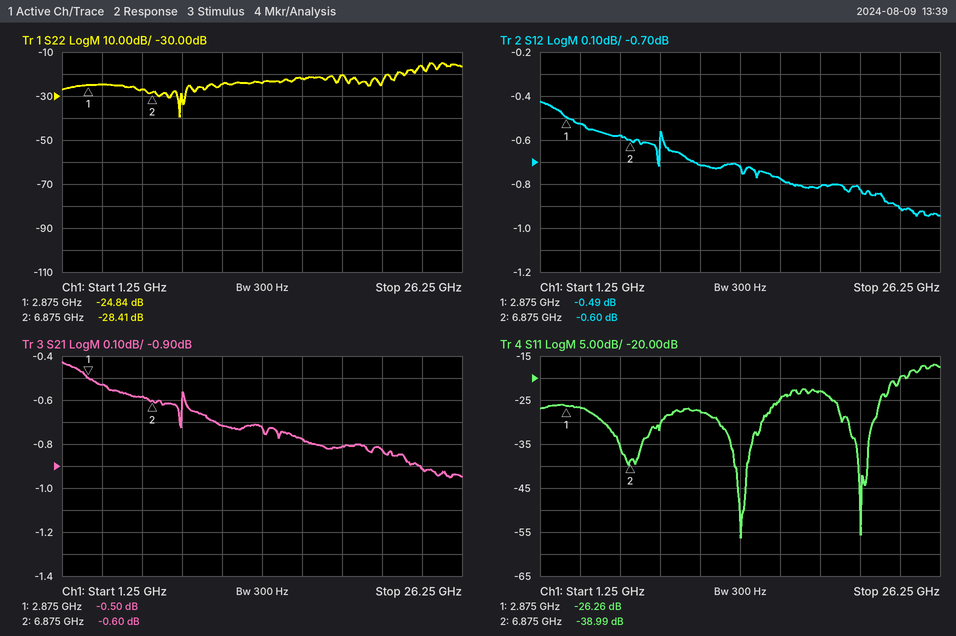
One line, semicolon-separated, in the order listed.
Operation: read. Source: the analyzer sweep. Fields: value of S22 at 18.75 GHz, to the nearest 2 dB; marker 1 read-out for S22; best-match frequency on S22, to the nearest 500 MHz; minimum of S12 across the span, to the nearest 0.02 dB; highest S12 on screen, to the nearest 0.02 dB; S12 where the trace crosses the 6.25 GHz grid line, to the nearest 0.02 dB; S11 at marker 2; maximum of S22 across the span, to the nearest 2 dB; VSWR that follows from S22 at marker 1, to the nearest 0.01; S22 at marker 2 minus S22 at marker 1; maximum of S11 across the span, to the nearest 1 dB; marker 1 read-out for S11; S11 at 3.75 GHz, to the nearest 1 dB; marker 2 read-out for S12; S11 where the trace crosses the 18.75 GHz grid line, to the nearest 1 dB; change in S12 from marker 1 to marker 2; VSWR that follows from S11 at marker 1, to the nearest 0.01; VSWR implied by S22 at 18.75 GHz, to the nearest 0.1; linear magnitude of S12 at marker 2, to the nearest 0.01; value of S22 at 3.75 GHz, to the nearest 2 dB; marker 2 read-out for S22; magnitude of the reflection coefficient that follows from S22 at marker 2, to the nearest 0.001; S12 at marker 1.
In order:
-20 dB; -24.84 dB; 8.5 GHz; -0.94 dB; -0.42 dB; -0.58 dB; -38.99 dB; -14 dB; 1.12; -3.57 dB; -17 dB; -26.26 dB; -27 dB; -0.60 dB; -23 dB; -0.11 dB; 1.10; 1.2; 0.93; -24 dB; -28.41 dB; 0.038; -0.49 dB
